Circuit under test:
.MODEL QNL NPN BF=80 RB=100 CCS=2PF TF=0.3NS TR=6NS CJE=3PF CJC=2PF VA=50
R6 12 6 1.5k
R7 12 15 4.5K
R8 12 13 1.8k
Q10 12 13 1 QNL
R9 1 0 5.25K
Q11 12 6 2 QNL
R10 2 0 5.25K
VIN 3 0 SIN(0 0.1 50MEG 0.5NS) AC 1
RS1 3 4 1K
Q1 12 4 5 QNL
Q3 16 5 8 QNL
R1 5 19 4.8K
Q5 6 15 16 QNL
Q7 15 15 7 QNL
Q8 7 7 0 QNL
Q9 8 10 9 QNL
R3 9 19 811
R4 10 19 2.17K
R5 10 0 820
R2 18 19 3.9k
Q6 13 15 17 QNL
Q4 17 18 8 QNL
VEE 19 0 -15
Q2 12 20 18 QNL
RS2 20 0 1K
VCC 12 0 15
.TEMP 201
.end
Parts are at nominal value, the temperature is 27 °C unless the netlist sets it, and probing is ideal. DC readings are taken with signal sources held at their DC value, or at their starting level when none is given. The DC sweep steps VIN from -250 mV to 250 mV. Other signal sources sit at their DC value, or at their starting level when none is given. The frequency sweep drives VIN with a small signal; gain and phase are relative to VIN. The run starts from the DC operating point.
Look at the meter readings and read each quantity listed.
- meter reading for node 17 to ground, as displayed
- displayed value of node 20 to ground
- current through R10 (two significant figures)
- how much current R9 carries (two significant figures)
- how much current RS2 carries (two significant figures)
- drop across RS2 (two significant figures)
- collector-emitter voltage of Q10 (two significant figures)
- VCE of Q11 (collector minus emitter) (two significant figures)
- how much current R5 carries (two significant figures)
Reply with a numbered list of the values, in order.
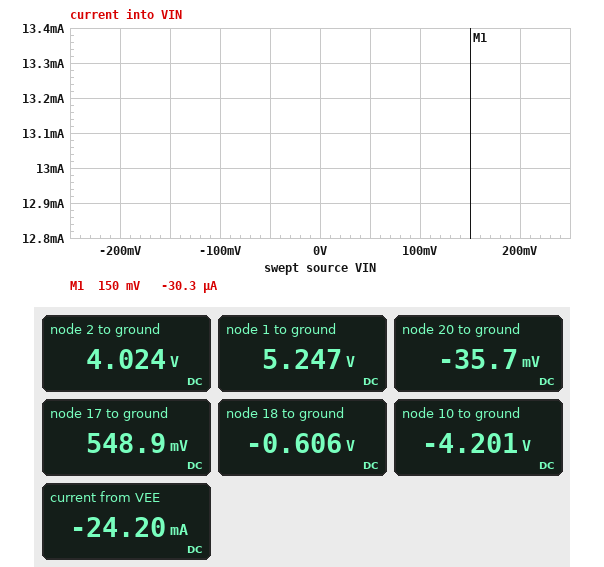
1. 548.9 mV
2. -35.7 mV
3. 770 µA
4. 1.0 mA
5. 36 µA
6. 36 mV
7. 9.8 V
8. 11 V
9. 5.1 mA
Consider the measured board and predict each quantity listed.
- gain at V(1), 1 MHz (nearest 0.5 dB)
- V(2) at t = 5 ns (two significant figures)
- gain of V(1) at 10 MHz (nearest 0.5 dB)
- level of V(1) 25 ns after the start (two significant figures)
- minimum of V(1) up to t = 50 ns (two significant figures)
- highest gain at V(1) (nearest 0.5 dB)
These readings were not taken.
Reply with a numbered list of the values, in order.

1. 40.5 dB
2. 3.9 V
3. 39.5 dB
4. 4.2 V
5. 3.7 V
6. 40.5 dB
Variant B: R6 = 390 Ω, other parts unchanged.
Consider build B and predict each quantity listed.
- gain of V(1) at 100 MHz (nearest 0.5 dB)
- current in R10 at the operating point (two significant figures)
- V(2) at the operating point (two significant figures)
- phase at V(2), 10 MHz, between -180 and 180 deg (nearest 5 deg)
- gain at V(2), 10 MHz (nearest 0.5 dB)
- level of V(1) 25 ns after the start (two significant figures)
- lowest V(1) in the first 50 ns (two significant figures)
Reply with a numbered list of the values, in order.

1. 7.0 dB
2. 2.2 mA
3. 12 V
4. 145 deg
5. 27.0 dB
6. 4.1 V
7. 3.6 V
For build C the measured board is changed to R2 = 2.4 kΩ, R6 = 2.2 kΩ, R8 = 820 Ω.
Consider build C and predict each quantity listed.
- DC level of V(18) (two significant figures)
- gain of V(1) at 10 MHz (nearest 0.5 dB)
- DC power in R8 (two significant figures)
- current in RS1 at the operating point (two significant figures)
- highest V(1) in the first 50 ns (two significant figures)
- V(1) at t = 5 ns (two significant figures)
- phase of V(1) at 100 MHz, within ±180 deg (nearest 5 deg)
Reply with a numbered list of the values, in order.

1. -650 mV
2. 31.0 dB
3. 6.6 mW
4. 30 µA
5. 14 V
6. 12 V
7. 130 deg
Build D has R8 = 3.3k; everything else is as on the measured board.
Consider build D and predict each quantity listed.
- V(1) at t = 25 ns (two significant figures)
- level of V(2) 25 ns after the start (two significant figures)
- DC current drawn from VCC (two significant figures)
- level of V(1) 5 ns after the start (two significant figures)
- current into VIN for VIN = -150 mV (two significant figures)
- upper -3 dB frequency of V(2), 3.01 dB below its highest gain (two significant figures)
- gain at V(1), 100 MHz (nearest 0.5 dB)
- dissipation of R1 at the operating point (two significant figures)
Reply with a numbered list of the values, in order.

1. -76 mV
2. 5.0 V
3. 22 mA
4. 210 mV
5. -29 µA
6. 19 MHz
7. -4.0 dB
8. 43 mW
